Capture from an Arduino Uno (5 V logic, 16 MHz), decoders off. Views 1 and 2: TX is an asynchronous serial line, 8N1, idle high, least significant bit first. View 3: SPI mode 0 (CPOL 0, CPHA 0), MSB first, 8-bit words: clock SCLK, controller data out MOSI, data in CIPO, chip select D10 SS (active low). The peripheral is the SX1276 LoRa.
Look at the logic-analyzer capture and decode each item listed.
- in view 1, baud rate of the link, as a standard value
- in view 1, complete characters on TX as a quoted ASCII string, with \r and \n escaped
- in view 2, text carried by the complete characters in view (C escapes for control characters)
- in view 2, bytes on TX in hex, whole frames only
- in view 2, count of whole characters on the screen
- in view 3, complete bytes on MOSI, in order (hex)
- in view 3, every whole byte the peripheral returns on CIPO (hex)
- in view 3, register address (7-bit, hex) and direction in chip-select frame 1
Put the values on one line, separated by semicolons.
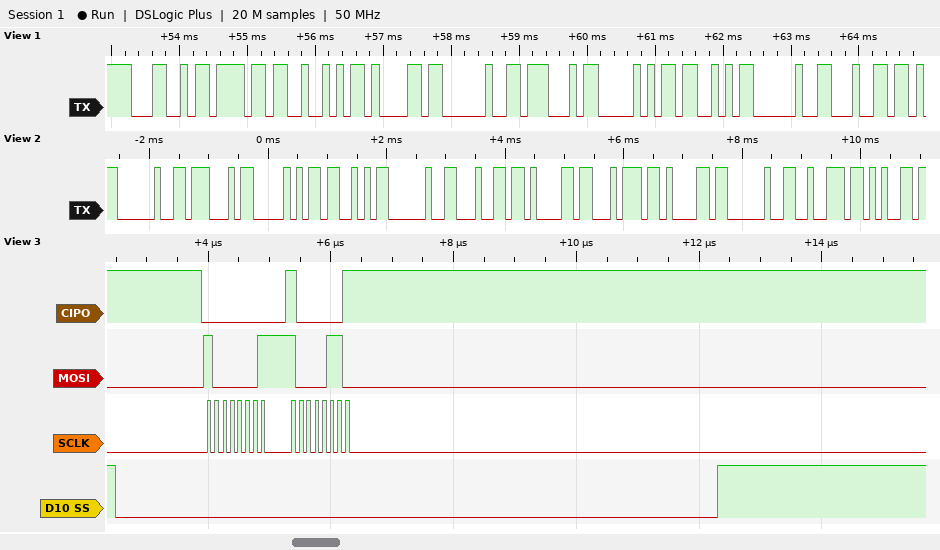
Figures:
9600 baud; "LoRa GPS d"; " GPS data re"; 0x20 0x47 0x50 0x53 0x20 0x64 0x61 0x74 0x61 0x20 0x72 0x65; 12; 0x81 0x86; 0x00 0x81; 0x01 write
